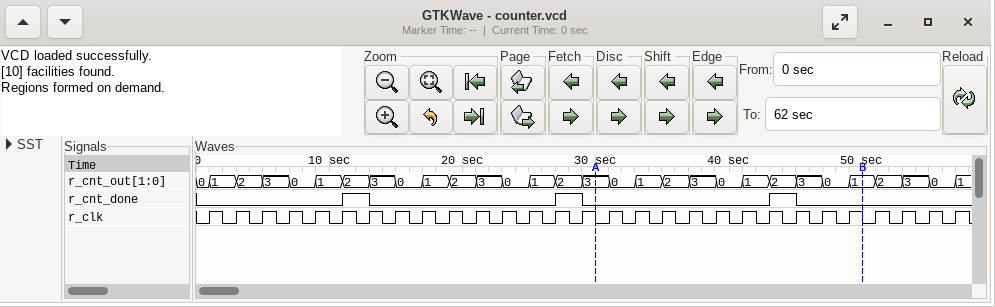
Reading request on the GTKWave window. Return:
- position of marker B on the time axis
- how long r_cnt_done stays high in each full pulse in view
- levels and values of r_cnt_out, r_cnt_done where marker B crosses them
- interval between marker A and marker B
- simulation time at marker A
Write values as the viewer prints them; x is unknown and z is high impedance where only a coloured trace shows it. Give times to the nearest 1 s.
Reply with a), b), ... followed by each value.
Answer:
a) 50 s
b) 2 s, 2 s, 2 s
c) r_cnt_out=1, r_cnt_done=0
d) 20 s
e) 30 s
